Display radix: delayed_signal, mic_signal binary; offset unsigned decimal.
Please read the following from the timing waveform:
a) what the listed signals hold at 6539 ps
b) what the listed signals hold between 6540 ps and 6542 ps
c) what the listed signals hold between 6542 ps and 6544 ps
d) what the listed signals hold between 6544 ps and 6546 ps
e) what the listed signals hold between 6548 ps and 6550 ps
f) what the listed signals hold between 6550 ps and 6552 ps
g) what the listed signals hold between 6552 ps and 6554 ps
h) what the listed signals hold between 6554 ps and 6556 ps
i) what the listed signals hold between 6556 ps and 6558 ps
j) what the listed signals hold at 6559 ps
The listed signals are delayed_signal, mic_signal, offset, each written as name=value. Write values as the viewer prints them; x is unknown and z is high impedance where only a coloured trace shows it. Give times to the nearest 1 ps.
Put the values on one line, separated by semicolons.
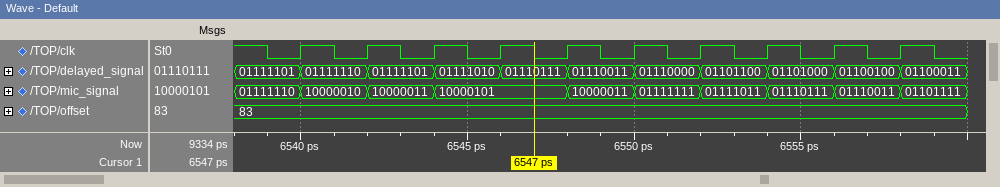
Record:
delayed_signal=01111101, mic_signal=01111110, offset=83; delayed_signal=01111110, mic_signal=10000010, offset=83; delayed_signal=01111101, mic_signal=10000011, offset=83; delayed_signal=01111010, mic_signal=10000101, offset=83; delayed_signal=01110011, mic_signal=10000011, offset=83; delayed_signal=01110000, mic_signal=01111111, offset=83; delayed_signal=01101100, mic_signal=01111011, offset=83; delayed_signal=01101000, mic_signal=01110111, offset=83; delayed_signal=01100100, mic_signal=01110011, offset=83; delayed_signal=01100011, mic_signal=01101111, offset=83
